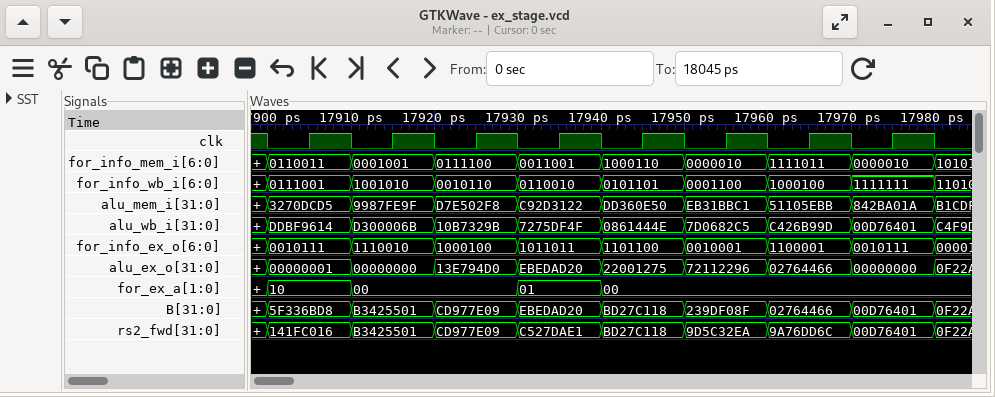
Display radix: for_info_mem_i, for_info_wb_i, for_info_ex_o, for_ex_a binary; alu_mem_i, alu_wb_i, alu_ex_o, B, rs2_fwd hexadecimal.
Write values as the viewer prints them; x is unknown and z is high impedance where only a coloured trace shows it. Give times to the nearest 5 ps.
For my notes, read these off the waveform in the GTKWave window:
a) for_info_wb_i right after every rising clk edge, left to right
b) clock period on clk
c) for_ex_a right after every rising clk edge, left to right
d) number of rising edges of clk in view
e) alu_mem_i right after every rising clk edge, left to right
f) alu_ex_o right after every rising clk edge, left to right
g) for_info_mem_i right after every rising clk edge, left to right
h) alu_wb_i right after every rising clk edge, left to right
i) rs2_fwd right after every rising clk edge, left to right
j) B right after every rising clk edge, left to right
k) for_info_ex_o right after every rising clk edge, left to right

0111001, 1001010, 0010110, 0110010, 0101101, 0001100, 1000100, 1111111
10 ps
10, 00, 00, 01, 00, 00, 00, 00
8
3270DCD5, 9987FE9F, D7E502F8, C92D3122, DD360E50, EB31BBC1, 51105EBB, 842BA01A
00000001, 00000000, 13E794D0, EBEDAD20, 22001275, 72112296, 02764466, 00000000
0110011, 0001001, 0111100, 0011001, 1000110, 0000010, 1111011, 0000010
DDBF9614, D300006B, 10B7329B, 7275DF4F, 0861444E, 7D0682C5, C426B99D, 00D76401
141FC016, B3425501, CD977E09, C527DAE1, BD27C118, 9D5C32EA, 9A76DD6C, 00D76401
5F336BD8, B3425501, CD977E09, EBEDAD20, BD27C118, 239DF08F, 02764466, 00D76401
0010111, 1110010, 1000100, 1011011, 1101100, 0010001, 1100001, 0010111
